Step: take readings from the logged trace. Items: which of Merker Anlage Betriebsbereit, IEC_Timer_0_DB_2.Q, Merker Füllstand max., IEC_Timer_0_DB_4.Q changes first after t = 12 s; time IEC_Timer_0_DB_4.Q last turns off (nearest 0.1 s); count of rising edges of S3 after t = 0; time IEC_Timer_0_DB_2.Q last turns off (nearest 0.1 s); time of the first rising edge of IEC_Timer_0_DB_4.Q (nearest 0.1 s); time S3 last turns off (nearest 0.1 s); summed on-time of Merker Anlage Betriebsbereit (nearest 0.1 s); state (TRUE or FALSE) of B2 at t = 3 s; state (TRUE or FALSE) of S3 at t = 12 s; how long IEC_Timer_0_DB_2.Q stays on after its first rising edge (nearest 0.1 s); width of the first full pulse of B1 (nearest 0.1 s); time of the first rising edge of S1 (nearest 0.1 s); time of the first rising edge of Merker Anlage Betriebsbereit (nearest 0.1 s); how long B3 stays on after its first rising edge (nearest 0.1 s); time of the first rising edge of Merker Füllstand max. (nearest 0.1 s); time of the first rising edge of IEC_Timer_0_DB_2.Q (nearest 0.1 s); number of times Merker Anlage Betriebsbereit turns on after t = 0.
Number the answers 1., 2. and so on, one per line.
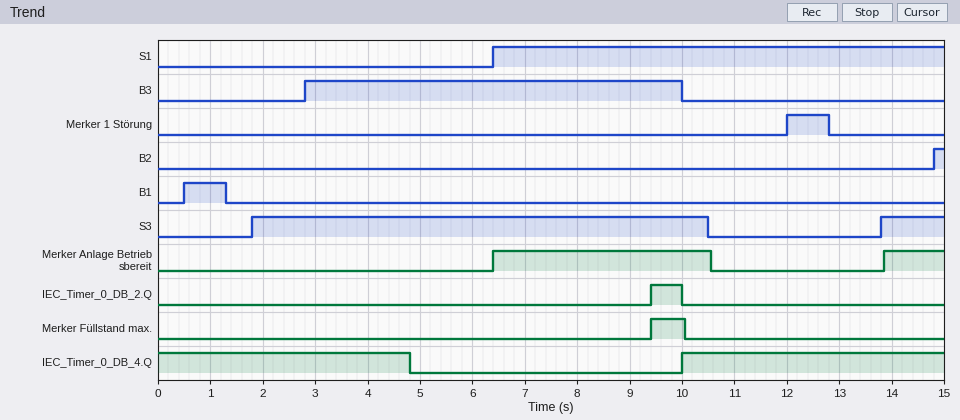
1. Merker Anlage Betriebsbereit
2. 4.8 s
3. 2
4. 10.0 s
5. 10.0 s
6. 10.5 s
7. 5.3 s
8. FALSE
9. FALSE
10. 0.6 s
11. 0.8 s
12. 6.4 s
13. 6.4 s
14. 7.2 s
15. 9.4 s
16. 9.4 s
17. 2
